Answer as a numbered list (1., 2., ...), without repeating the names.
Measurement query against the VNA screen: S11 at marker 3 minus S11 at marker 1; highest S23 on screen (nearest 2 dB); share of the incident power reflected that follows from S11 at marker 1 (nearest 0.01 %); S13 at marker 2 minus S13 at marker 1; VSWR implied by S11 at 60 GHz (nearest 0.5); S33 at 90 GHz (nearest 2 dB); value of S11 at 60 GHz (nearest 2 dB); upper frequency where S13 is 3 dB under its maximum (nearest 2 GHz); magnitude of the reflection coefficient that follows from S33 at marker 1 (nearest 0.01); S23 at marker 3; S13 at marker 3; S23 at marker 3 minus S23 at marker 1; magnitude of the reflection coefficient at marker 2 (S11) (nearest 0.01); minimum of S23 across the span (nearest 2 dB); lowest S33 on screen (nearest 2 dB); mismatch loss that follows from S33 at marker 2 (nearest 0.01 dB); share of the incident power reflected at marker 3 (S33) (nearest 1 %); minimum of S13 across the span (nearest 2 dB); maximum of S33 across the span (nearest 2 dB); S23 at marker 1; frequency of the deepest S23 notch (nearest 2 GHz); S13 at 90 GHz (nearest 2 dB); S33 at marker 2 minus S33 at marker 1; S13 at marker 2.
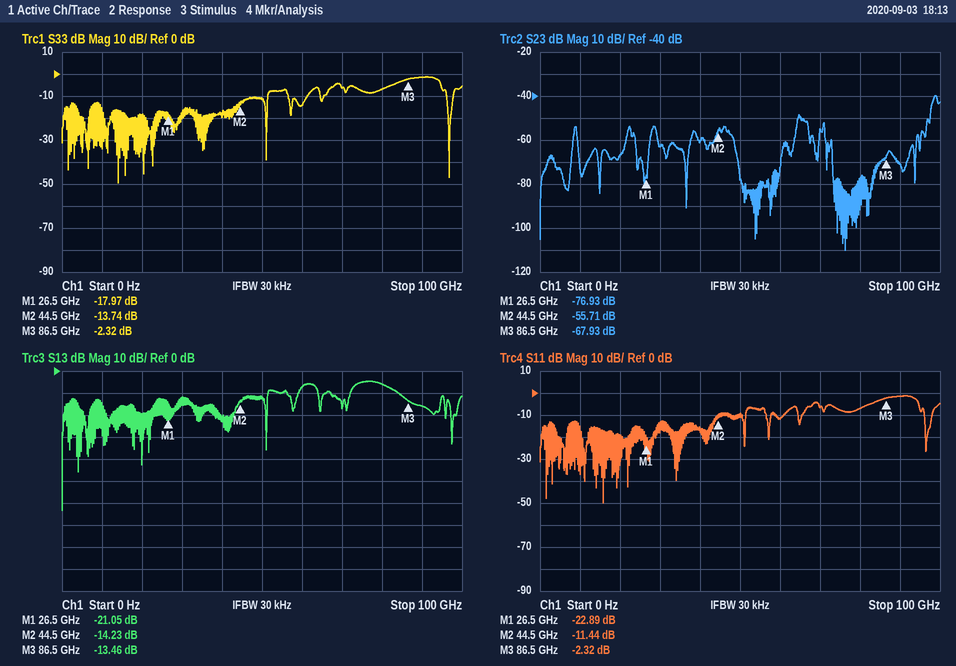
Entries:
1. 20.57 dB
2. -40 dB
3. 0.51 %
4. 6.82 dB
5. 1.5
6. -2 dB
7. -12 dB
8. 82 GHz
9. 0.13
10. -67.93 dB
11. -13.46 dB
12. 9.00 dB
13. 0.27
14. -110 dB
15. -50 dB
16. 0.19 dB
17. 59 %
18. -64 dB
19. -2 dB
20. -76.93 dB
21. 76 GHz
22. -16 dB
23. 4.23 dB
24. -14.23 dB
